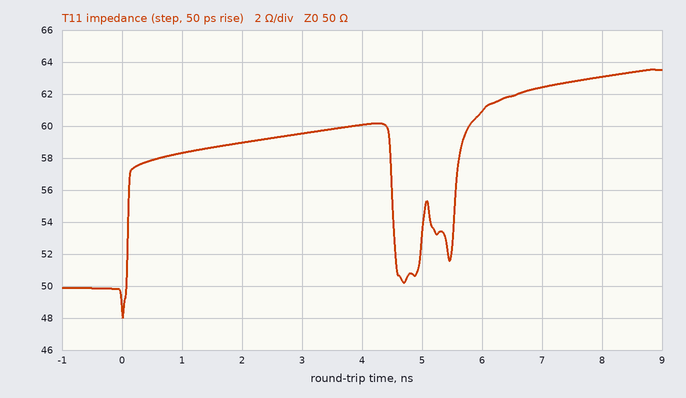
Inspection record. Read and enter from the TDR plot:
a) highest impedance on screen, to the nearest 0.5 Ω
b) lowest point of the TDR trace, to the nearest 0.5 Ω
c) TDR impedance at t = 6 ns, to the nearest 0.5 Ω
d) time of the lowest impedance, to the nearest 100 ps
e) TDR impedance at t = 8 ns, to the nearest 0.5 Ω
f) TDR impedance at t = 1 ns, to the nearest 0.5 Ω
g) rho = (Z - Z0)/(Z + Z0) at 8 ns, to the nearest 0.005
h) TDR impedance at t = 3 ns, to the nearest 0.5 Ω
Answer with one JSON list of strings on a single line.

["63.5 Ω", "48.0 Ω", "61.0 Ω", "0.0 ns", "63.0 Ω", "58.5 Ω", "+0.115", "59.5 Ω"]
